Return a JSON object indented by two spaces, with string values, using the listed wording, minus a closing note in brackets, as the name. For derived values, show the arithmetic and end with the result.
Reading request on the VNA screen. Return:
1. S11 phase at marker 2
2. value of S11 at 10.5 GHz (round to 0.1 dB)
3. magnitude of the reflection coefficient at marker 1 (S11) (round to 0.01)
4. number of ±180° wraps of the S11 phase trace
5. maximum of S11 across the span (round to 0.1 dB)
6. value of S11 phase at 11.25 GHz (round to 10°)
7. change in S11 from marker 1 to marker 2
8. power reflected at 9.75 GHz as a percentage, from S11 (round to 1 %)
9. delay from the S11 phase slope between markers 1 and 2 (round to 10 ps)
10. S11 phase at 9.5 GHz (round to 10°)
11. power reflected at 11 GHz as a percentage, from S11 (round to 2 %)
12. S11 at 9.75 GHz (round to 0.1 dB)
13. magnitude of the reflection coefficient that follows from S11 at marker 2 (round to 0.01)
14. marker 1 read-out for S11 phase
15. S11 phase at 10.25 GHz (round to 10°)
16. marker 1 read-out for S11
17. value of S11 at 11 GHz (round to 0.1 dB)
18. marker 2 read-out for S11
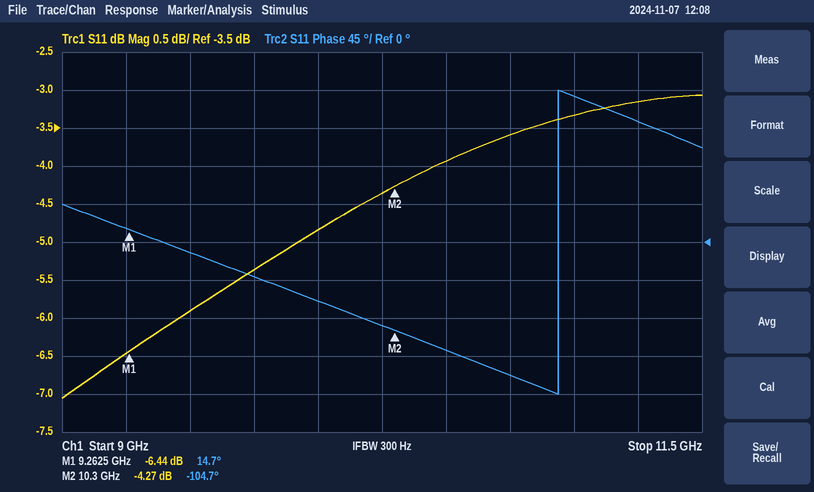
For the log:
{
  "S11 phase at marker 2": "-104.7°",
  "value of S11 at 10.5 GHz": "-3.9 dB",
  "magnitude of the reflection coefficient at marker 1 (S11)": "10^(-6.44/20) ≈ 0.48",
  "number of ±180° wraps of the S11 phase trace": "1",
  "maximum of S11 across the span": "-3.1 dB",
  "value of S11 phase at 11.25 GHz": "140°",
  "change in S11 from marker 1 to marker 2": "-4.27 − (-6.44) = 2.17 dB",
  "power reflected at 9.75 GHz as a percentage, from S11": "10^(-5.4/10) ≈ 29 %",
  "delay from the S11 phase slope between markers 1 and 2": "−(-104.7° − (14.7°))/(360° × 1.0375 GHz) ≈ 320 ps",
  "S11 phase at 9.5 GHz": "-10°",
  "power reflected at 11 GHz as a percentage, from S11": "10^(-3.3/10) ≈ 46.8 %, so 46 % to the nearest 2 %",
  "S11 at 9.75 GHz": "-5.4 dB",
  "magnitude of the reflection coefficient that follows from S11 at marker 2": "10^(-4.27/20) ≈ 0.61",
  "marker 1 read-out for S11 phase": "14.7°",
  "S11 phase at 10.25 GHz": "-100°",
  "marker 1 read-out for S11": "-6.44 dB",
  "value of S11 at 11 GHz": "-3.3 dB",
  "marker 2 read-out for S11": "-4.27 dB"
}
